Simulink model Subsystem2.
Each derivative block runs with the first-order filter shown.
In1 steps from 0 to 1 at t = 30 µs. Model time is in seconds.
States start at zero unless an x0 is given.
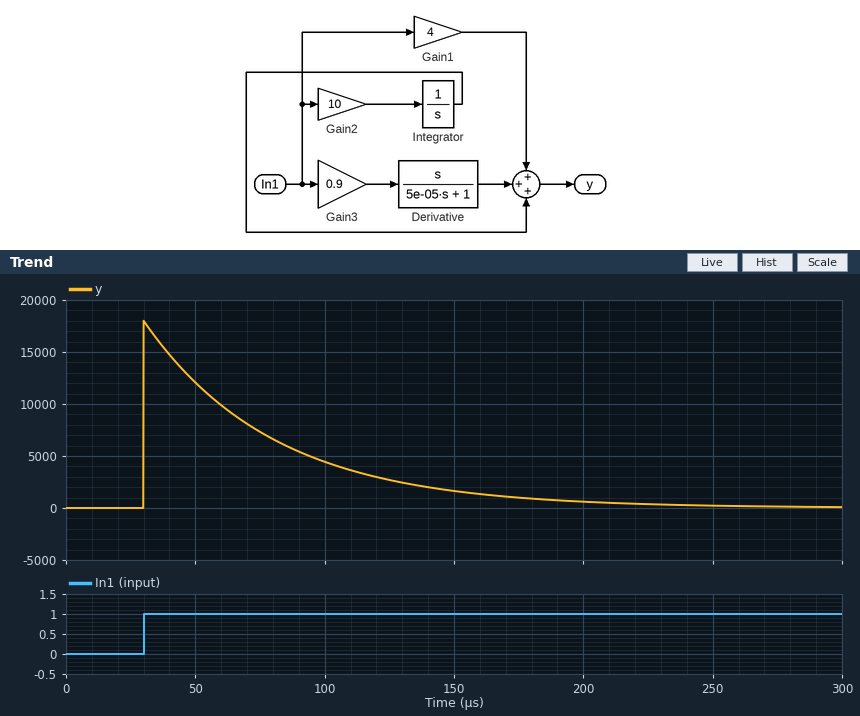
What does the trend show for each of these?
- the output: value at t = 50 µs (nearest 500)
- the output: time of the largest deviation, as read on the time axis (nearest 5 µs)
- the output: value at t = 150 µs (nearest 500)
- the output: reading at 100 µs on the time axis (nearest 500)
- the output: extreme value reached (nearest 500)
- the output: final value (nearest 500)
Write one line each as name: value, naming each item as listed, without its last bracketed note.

the output: value at t = 50 µs: 12000
the output: time of the largest deviation, as read on the time axis: 30 µs
the output: value at t = 150 µs: 1500
the output: reading at 100 µs on the time axis: 4500
the output: extreme value reached: 18000
the output: final value: 0
